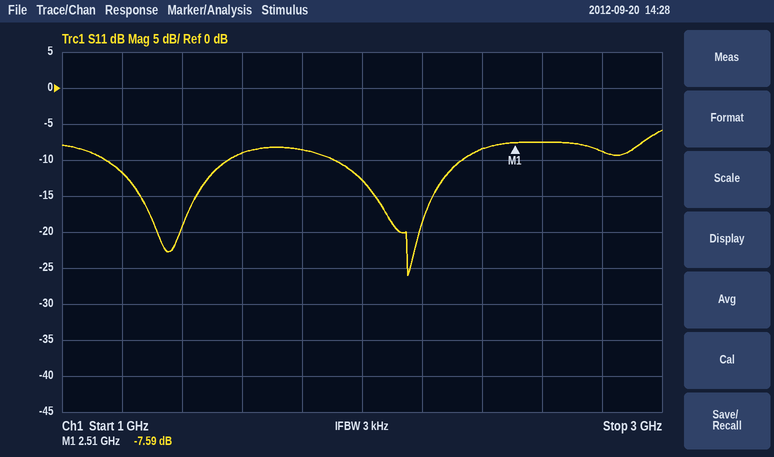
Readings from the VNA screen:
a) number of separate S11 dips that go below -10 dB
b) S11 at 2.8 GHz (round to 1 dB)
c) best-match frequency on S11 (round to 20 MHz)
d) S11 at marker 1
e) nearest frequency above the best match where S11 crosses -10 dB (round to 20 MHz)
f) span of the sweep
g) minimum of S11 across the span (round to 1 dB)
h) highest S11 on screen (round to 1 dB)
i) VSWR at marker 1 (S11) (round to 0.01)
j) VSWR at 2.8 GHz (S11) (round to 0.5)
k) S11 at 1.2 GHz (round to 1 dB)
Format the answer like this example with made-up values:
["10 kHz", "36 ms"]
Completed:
["2", "-9 dB", "2.16 GHz", "-7.59 dB", "2.34 GHz", "2 GHz", "-26 dB", "-6 dB", "2.43", "2.0", "-12 dB"]
